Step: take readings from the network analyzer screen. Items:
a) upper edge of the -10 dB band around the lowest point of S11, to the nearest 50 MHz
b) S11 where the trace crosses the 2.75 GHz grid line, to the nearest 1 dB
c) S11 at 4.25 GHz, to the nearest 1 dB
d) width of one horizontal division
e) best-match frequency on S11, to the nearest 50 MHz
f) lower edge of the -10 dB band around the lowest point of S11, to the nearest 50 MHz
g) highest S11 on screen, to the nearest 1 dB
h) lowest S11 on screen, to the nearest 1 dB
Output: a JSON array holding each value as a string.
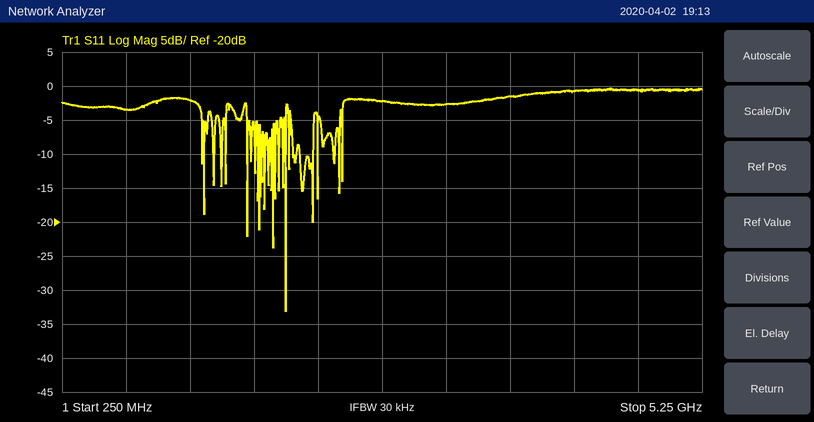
["2.00 GHz", "-2 dB", "-1 dB", "500 MHz", "2.00 GHz", "2.00 GHz", "0 dB", "-33 dB"]
